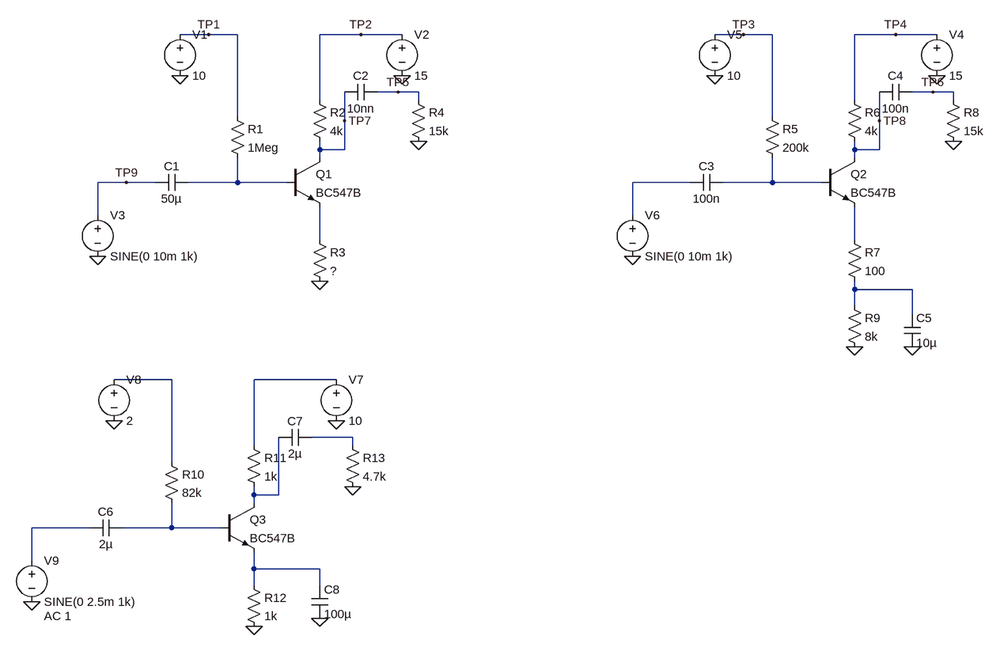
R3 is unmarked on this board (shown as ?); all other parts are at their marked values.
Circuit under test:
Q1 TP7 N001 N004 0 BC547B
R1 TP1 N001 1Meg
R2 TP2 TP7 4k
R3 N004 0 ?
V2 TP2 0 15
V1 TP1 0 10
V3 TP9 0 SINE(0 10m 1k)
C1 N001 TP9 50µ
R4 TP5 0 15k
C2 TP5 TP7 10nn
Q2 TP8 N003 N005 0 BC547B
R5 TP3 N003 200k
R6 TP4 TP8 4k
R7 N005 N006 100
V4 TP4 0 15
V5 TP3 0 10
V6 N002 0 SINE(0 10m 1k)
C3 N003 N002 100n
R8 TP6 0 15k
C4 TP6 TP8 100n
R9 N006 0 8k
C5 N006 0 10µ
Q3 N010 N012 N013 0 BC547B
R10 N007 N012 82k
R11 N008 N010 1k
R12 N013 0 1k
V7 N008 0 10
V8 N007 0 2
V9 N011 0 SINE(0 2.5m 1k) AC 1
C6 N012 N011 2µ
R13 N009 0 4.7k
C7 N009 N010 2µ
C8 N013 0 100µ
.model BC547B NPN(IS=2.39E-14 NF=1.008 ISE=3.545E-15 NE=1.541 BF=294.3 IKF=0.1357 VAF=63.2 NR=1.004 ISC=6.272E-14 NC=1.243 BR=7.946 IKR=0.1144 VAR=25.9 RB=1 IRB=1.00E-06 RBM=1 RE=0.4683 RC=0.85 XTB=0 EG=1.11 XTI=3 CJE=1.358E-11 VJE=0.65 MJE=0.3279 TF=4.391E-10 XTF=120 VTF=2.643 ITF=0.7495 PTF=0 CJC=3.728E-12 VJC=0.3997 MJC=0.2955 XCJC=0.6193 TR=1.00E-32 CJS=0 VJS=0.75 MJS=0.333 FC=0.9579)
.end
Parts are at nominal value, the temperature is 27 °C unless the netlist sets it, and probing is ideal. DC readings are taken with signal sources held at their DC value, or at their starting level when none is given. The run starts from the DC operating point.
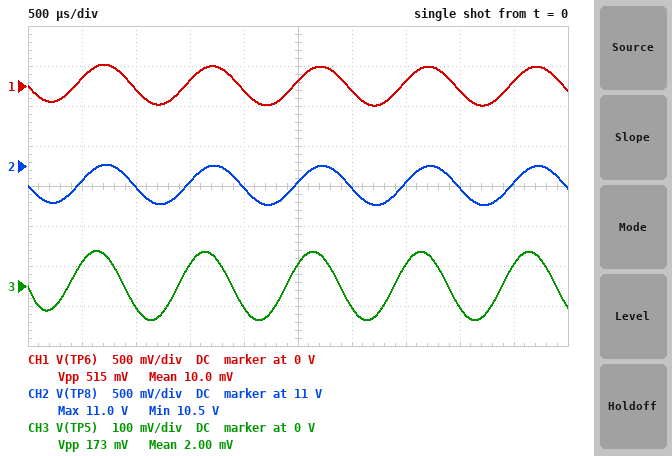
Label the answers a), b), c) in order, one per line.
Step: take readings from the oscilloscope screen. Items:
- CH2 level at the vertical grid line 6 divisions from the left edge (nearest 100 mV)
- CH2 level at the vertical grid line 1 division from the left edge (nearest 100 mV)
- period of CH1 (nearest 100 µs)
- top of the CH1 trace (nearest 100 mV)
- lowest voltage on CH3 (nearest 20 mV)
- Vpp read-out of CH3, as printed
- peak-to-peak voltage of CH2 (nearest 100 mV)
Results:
a) 10.7 V
b) 10.8 V
c) 1.0 ms
d) 300 mV
e) -80 mV
f) 173 mV
g) 500 mV
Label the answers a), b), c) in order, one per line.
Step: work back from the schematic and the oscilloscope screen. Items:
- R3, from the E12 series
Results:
a) 270 Ω
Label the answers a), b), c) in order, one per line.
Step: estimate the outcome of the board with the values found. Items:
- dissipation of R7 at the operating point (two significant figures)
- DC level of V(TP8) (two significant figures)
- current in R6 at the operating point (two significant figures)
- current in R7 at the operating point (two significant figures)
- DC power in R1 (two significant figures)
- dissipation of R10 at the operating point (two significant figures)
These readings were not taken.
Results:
a) 110 µW
b) 11 V
c) 1.1 mA
d) 1.1 mA
e) 75 µW
f) 960 nW
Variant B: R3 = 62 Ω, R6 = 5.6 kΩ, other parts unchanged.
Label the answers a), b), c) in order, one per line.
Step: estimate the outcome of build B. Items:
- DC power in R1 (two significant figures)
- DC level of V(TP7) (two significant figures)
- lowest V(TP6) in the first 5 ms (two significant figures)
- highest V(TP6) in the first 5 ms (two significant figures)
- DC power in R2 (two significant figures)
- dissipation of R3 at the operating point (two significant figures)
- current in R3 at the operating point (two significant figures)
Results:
a) 84 µW
b) 4.2 V
c) -310 mV
d) 350 mV
e) 29 mW
f) 460 µW
g) 2.7 mA
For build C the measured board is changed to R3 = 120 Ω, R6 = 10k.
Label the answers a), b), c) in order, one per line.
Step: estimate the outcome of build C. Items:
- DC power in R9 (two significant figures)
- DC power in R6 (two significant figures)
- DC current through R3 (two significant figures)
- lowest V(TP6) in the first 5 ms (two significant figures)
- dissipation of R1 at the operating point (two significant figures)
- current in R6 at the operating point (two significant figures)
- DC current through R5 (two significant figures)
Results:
a) 5.5 mW
b) 6.7 mW
c) 2.7 mA
d) -13 mV
e) 81 µW
f) 820 µA
g) 13 µA
